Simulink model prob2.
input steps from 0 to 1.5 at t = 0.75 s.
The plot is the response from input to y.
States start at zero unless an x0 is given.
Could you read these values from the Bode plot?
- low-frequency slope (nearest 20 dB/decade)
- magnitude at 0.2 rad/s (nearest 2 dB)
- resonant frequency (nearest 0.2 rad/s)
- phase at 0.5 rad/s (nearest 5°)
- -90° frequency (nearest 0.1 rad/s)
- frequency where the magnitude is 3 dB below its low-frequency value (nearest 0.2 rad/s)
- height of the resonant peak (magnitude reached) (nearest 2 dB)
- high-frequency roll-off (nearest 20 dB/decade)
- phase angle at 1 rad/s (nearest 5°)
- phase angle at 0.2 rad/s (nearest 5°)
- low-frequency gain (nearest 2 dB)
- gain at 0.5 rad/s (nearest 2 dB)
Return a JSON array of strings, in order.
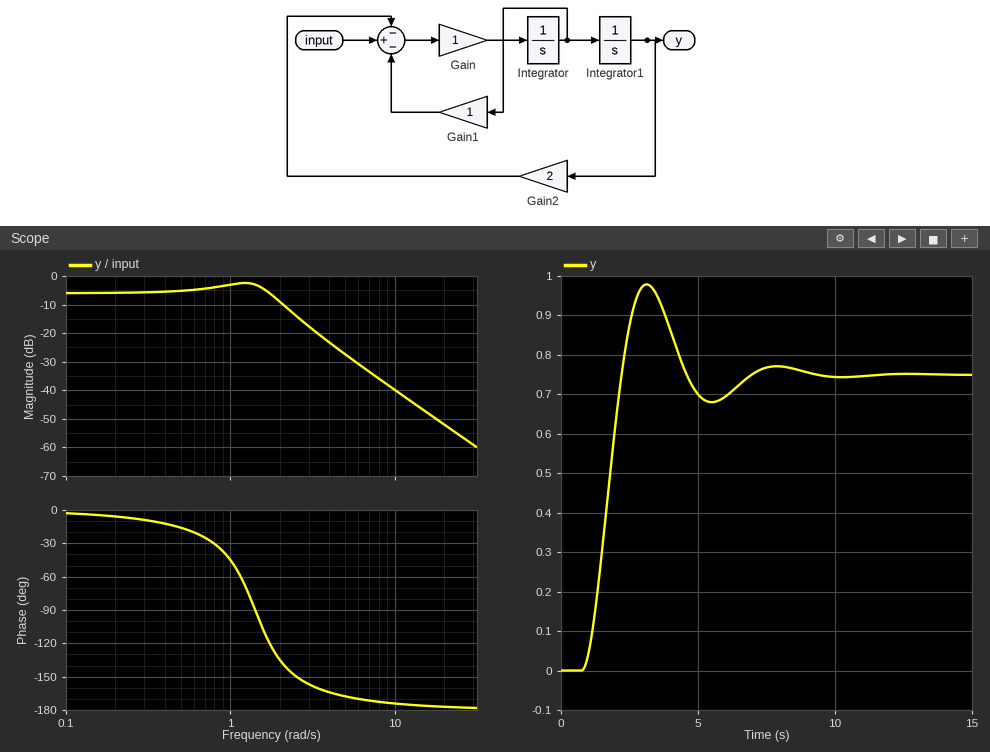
["0 dB/decade", "-6 dB", "1.2 rad/s", "-15°", "1.4 rad/s", "2.0 rad/s", "-2 dB", "-40 dB/decade", "-45°", "-5°", "-6 dB", "-6 dB"]
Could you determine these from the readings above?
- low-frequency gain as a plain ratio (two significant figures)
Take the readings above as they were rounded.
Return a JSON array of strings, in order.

["0.50"]
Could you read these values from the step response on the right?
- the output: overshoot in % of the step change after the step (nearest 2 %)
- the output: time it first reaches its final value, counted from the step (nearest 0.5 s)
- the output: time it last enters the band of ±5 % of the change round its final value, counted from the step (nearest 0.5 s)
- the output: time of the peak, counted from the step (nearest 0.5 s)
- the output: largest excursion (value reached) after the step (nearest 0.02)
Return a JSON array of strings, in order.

["30 %", "1.5 s", "5.5 s", "2.5 s", "0.98"]
